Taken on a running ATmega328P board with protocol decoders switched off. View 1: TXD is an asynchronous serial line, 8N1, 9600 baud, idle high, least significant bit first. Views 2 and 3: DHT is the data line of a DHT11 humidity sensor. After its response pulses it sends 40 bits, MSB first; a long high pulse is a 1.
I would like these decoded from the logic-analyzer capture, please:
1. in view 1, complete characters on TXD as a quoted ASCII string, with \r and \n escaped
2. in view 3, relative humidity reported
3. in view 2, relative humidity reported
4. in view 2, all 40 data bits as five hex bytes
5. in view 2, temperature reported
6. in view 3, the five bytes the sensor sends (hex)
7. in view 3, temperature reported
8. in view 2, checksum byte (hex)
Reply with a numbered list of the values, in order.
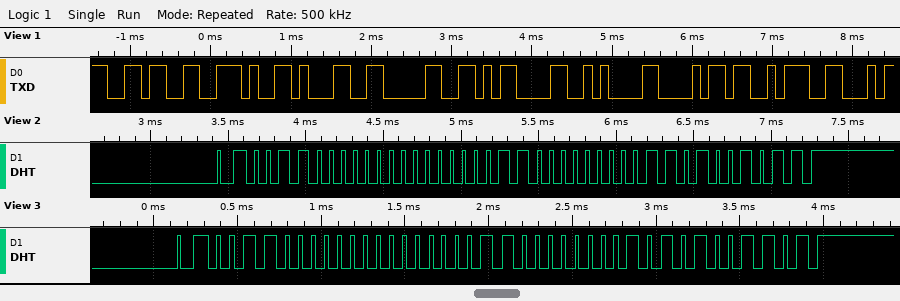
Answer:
1. "6.10\r\nh:"
2. 48 %
3. 48 %
4. 30 00 18 03 4B
5. 24.3 °C
6. 30 00 18 05 4D
7. 24.5 °C
8. 0x4B
